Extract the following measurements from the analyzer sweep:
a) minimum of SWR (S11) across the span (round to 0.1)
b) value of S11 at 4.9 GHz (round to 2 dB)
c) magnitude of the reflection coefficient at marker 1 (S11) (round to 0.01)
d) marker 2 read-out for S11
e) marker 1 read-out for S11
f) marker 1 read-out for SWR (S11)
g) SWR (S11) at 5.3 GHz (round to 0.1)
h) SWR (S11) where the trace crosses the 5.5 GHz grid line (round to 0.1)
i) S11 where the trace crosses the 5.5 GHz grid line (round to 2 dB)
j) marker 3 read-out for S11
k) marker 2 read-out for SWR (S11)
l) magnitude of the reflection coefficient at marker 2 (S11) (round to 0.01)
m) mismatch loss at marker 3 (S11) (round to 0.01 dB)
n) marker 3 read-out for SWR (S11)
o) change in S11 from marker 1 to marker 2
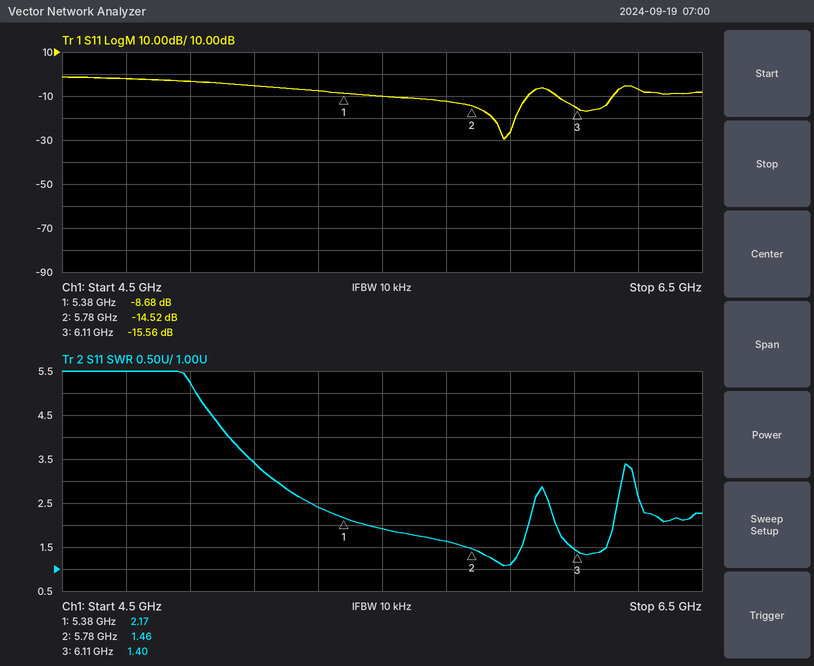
1.1
-4 dB
0.37
-14.52 dB
-8.68 dB
2.17
2.4
1.9
-10 dB
-15.56 dB
1.46
0.19
0.12 dB
1.40
-5.84 dB
